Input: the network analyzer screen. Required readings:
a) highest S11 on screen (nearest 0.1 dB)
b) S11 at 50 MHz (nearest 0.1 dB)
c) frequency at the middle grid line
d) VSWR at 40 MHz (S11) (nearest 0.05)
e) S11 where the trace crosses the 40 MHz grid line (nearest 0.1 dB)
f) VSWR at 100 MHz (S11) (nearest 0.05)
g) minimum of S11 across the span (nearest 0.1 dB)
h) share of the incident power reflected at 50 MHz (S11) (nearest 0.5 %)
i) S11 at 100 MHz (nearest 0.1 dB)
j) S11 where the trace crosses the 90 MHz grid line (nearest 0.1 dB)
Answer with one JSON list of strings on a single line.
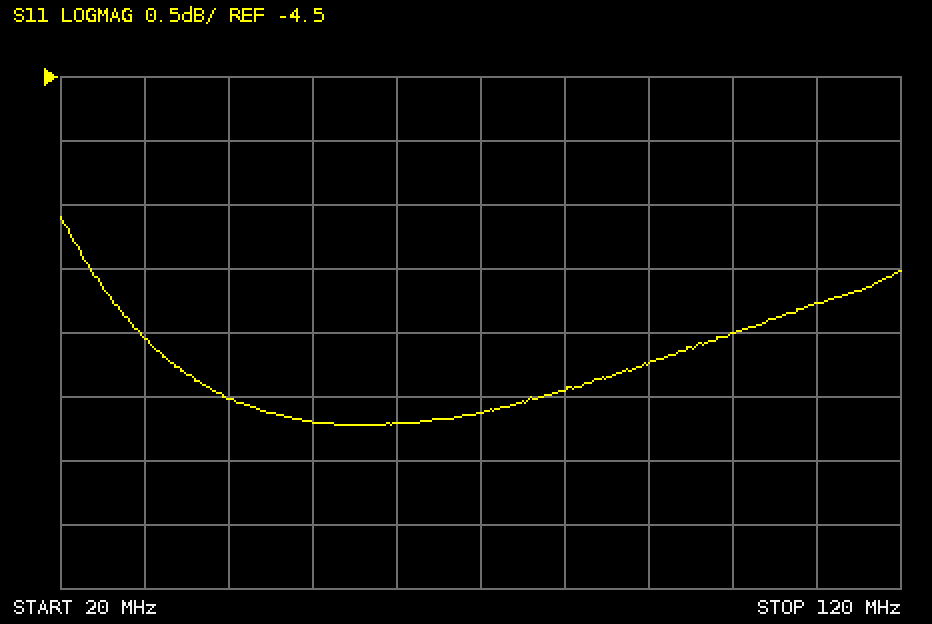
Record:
["-5.6 dB", "-7.2 dB", "70 MHz", "2.60", "-7.0 dB", "2.80", "-7.2 dB", "19.0 %", "-6.5 dB", "-6.7 dB"]
